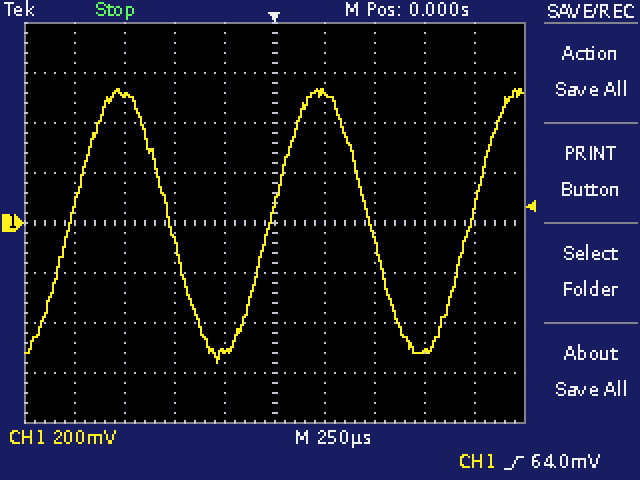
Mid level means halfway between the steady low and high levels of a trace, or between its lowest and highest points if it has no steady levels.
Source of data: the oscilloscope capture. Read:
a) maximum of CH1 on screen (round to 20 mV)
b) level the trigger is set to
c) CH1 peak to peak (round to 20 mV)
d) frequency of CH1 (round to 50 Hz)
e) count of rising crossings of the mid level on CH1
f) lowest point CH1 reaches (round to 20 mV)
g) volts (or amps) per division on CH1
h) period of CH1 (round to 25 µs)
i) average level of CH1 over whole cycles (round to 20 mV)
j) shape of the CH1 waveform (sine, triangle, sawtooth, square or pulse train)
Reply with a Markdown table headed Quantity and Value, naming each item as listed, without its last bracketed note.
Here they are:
| Quantity | Value |
|---|---|
| maximum of CH1 on screen | 540 mV |
| level the trigger is set to | 64.0 mV |
| CH1 peak to peak | 1.10 V |
| frequency of CH1 | 1.00 kHz |
| count of rising crossings of the mid level on CH1 | 3 |
| lowest point CH1 reaches | -560 mV |
| volts (or amps) per division on CH1 | 200 mV |
| period of CH1 | 1.000 ms |
| average level of CH1 over whole cycles | 0 mV |
| shape of the CH1 waveform | sine |
